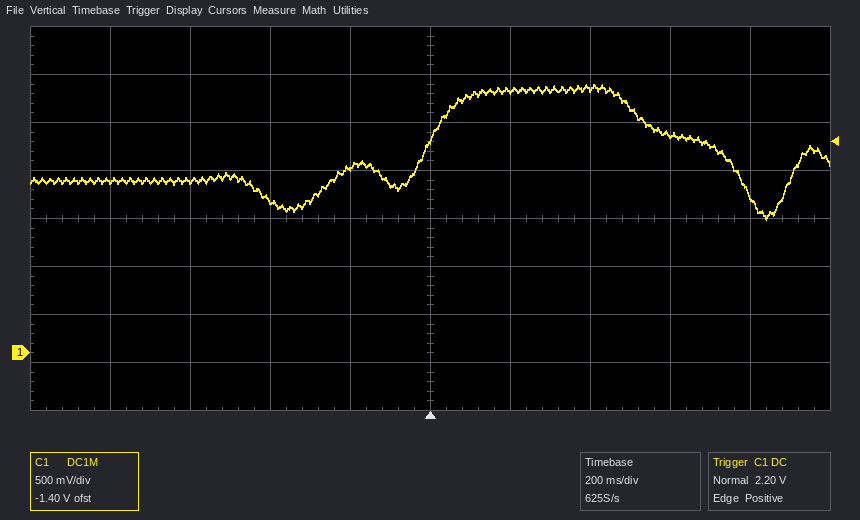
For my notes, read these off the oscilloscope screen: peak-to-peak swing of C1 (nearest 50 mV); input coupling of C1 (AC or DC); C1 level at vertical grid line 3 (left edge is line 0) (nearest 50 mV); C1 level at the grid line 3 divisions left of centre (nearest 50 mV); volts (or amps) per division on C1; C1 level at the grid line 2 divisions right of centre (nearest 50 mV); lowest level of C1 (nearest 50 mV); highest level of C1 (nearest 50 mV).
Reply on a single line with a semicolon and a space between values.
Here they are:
1.40 V; DC; 1.60 V; 1.80 V; 500 mV; 2.75 V; 1.40 V; 2.80 V
